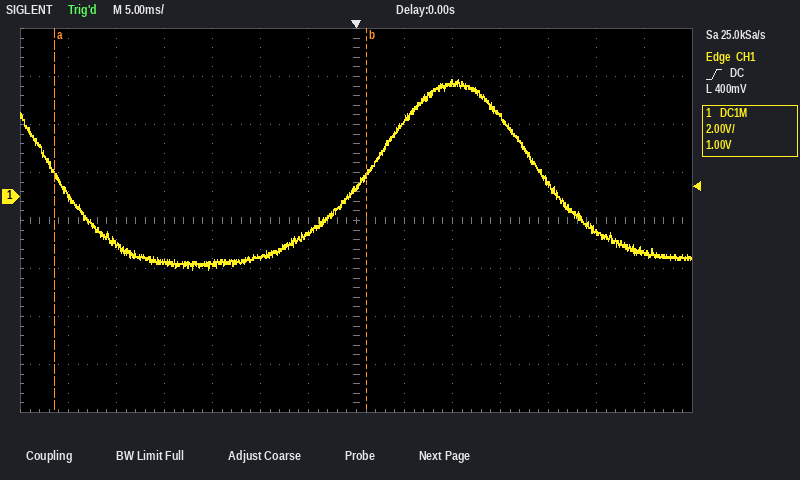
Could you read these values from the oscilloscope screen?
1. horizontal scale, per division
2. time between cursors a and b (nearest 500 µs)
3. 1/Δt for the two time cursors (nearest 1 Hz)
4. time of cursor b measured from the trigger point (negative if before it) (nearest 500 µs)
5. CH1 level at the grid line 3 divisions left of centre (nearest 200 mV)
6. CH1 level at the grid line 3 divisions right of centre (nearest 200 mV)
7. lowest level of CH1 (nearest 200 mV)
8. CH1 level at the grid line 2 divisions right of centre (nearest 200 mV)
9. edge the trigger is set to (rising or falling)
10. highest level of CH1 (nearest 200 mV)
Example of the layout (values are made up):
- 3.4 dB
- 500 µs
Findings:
- 5 ms
- 32.5 ms
- 31 Hz
- +1.0 ms
- -2.8 V
- 3.4 V
- -3.0 V
- 4.8 V
- rising
- 4.8 V
